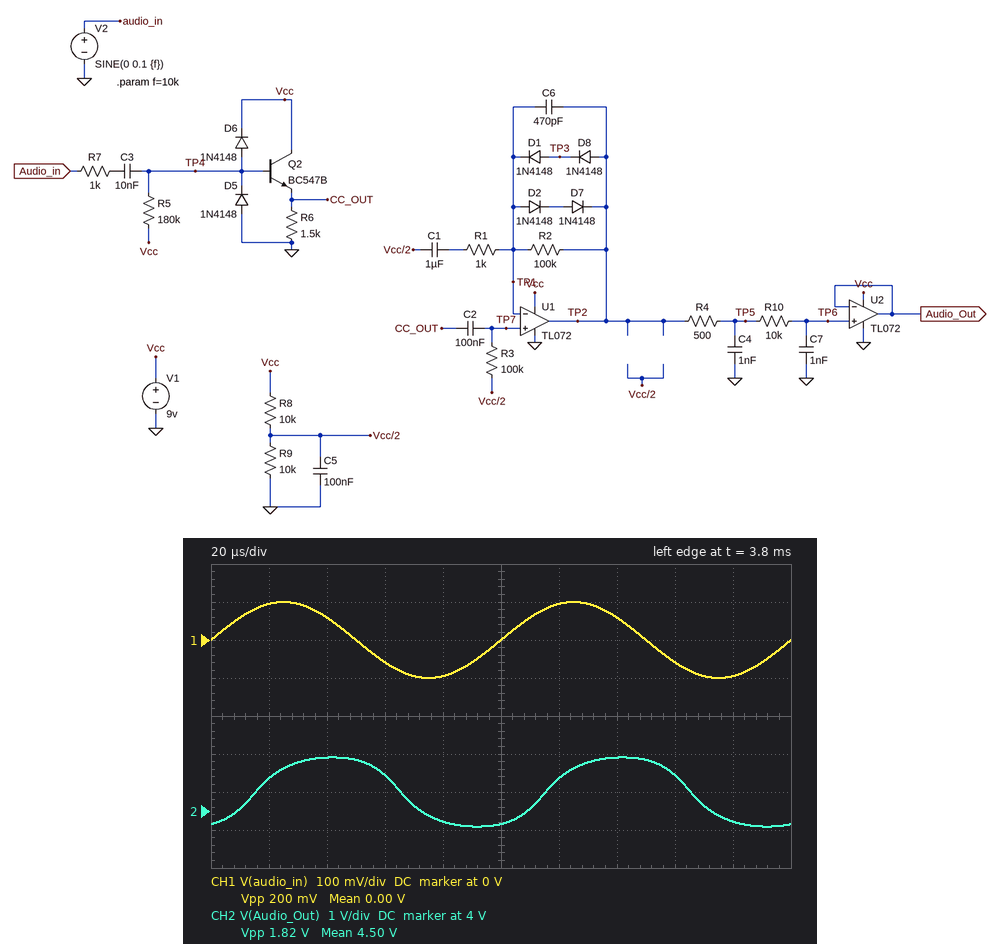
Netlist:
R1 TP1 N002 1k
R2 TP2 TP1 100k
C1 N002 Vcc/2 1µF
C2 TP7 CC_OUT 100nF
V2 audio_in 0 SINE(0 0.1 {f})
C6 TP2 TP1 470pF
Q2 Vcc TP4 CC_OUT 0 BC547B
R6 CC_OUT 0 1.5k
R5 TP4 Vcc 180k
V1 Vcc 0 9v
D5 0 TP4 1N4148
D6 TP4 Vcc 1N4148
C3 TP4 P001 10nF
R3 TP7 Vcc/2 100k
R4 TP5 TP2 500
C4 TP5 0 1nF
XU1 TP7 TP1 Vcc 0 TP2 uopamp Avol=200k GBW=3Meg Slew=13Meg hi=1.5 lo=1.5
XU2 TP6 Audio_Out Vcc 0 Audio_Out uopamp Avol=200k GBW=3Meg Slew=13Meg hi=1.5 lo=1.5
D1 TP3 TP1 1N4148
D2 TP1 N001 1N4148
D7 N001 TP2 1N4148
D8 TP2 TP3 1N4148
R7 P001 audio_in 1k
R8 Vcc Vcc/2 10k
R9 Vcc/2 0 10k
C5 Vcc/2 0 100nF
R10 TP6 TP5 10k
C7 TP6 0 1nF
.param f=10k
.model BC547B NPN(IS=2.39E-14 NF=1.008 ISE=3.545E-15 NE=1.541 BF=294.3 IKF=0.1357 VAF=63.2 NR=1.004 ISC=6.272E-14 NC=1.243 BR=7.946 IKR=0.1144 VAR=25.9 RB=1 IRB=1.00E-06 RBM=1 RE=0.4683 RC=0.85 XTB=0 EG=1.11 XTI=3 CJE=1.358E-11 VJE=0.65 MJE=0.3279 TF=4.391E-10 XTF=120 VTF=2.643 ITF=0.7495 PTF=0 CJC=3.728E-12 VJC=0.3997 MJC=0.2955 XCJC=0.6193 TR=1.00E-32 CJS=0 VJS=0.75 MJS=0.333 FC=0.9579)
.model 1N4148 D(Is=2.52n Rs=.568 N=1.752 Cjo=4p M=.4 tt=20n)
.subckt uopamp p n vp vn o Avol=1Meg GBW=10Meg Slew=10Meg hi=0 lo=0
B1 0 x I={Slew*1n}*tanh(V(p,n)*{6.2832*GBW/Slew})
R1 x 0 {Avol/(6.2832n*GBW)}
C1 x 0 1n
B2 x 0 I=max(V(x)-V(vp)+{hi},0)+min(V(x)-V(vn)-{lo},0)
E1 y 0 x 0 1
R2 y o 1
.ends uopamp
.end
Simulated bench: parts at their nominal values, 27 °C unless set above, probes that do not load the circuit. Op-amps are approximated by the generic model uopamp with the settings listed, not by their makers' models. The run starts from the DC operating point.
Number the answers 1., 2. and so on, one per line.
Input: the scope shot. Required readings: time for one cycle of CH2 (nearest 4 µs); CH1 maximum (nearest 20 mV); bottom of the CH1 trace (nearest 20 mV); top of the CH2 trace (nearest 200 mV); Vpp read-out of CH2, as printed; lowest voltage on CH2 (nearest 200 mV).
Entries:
1. 100 µs
2. 100 mV
3. -100 mV
4. 5.4 V
5. 1.82 V
6. 3.6 V
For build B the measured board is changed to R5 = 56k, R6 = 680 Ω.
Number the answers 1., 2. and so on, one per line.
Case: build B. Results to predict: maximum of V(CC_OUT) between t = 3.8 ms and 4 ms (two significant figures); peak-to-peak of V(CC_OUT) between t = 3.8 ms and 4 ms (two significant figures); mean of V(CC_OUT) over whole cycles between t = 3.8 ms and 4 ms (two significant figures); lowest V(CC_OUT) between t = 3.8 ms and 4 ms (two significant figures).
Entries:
1. 6.5 V
2. 190 mV
3. 6.4 V
4. 6.3 V
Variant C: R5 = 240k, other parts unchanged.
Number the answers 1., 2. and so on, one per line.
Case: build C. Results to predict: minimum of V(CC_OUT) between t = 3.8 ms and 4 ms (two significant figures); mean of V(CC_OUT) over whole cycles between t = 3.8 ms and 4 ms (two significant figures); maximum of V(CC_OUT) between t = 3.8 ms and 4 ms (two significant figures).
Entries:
1. 5.3 V
2. 5.4 V
3. 5.5 V
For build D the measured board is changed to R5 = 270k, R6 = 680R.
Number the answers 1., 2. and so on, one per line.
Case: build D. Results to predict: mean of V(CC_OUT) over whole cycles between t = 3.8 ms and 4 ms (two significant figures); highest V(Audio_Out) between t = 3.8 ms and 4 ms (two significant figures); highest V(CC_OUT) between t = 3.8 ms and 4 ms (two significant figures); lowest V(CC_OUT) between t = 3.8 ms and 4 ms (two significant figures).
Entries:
1. 3.6 V
2. 5.4 V
3. 3.7 V
4. 3.5 V
